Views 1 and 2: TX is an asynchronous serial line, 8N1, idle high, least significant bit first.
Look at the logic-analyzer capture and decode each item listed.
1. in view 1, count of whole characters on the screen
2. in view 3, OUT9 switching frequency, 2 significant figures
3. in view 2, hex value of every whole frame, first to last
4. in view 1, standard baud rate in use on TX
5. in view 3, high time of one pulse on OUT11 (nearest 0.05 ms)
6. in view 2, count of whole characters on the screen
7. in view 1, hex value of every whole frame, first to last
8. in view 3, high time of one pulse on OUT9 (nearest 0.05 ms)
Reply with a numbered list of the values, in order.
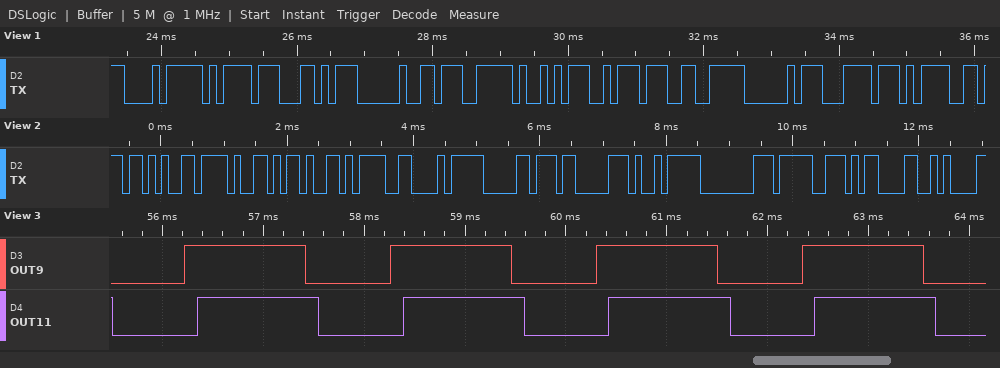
1. 11
2. 490 Hz
3. 0x2B 0x2F 0x2D 0x3D 0xE8 0xB0 0x83 0xE9 0x80 0x9F 0x0D 0x0A
4. 9600 baud
5. 1.20 ms
6. 12
7. E8 BD AC 20 E7 A9 BA E6 A0 BC 3D
8. 1.20 ms
